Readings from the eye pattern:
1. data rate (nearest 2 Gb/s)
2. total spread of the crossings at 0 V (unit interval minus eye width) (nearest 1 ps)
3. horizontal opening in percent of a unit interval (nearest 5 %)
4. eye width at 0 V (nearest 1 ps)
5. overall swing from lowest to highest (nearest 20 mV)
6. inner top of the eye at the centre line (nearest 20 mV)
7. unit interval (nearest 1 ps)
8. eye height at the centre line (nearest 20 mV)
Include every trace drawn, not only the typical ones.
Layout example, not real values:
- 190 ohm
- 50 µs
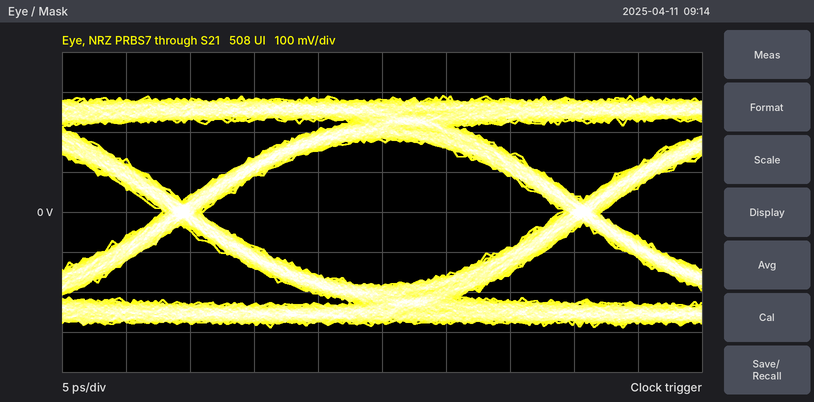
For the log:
- 32 Gb/s
- 3 ps
- 90 %
- 28 ps
- 580 mV
- 180 mV
- 31 ps
- 360 mV
